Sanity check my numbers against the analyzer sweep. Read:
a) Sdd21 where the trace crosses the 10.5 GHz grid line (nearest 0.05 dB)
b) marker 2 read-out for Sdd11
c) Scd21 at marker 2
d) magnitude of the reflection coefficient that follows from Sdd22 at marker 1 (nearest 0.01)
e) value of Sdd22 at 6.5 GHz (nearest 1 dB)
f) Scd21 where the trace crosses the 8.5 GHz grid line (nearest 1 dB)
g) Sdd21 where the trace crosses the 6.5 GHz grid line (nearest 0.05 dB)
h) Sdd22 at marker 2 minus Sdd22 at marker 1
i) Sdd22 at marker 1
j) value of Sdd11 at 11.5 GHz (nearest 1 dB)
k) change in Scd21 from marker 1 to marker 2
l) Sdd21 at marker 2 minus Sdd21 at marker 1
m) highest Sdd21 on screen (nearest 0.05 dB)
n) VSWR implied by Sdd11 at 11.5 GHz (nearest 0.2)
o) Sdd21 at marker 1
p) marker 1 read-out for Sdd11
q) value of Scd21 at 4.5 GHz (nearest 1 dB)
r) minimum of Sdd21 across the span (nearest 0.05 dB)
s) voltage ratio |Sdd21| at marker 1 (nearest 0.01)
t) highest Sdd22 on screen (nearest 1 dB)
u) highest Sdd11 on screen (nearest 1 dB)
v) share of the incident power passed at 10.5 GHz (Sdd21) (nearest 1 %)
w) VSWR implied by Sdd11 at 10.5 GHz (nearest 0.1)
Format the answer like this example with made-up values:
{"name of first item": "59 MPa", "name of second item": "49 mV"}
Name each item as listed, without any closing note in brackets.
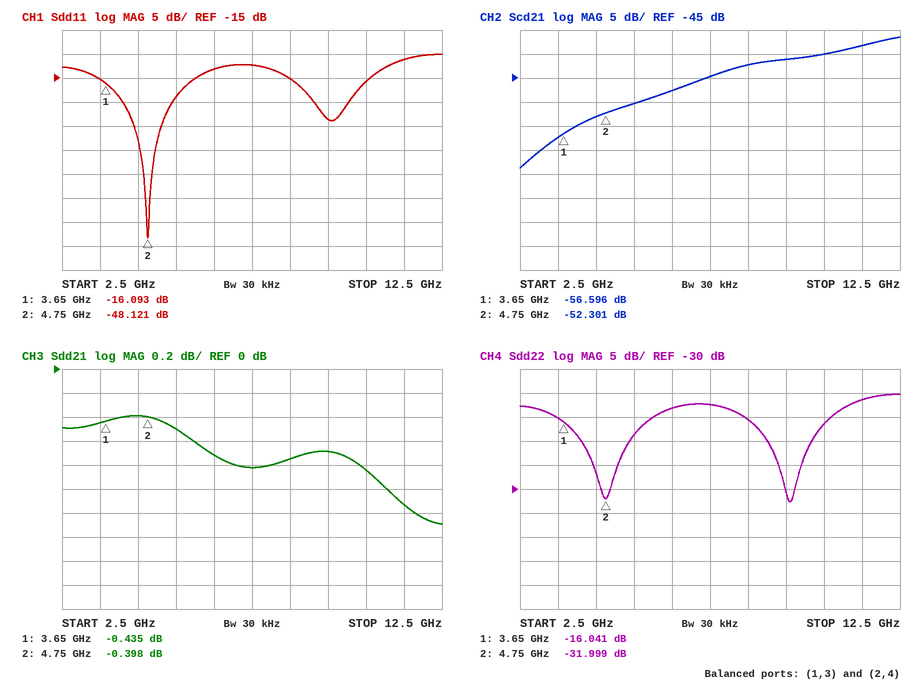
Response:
{"Sdd21 where the trace crosses the 10.5 GHz grid line": "-0.85 dB", "marker 2 read-out for Sdd11": "-48.121 dB", "Scd21 at marker 2": "-52.301 dB", "magnitude of the reflection coefficient that follows from Sdd22 at marker 1": "0.16", "value of Sdd22 at 6.5 GHz": "-13 dB", "Scd21 where the trace crosses the 8.5 GHz grid line": "-42 dB", "Sdd21 where the trace crosses the 6.5 GHz grid line": "-0.70 dB", "Sdd22 at marker 2 minus Sdd22 at marker 1": "-15.958 dB", "Sdd22 at marker 1": "-16.041 dB", "value of Sdd11 at 11.5 GHz": "-11 dB", "change in Scd21 from marker 1 to marker 2": "4.295 dB", "Sdd21 at marker 2 minus Sdd21 at marker 1": "0.037 dB", "highest Sdd21 on screen": "-0.40 dB", "VSWR implied by Sdd11 at 11.5 GHz": "1.8", "Sdd21 at marker 1": "-0.435 dB", "marker 1 read-out for Sdd11": "-16.093 dB", "value of Scd21 at 4.5 GHz": "-53 dB", "minimum of Sdd21 across the span": "-1.30 dB", "voltage ratio |Sdd21| at marker 1": "0.95", "highest Sdd22 on screen": "-10 dB", "highest Sdd11 on screen": "-10 dB", "share of the incident power passed at 10.5 GHz (Sdd21)": "82 %", "VSWR implied by Sdd11 at 10.5 GHz": "1.4"}
